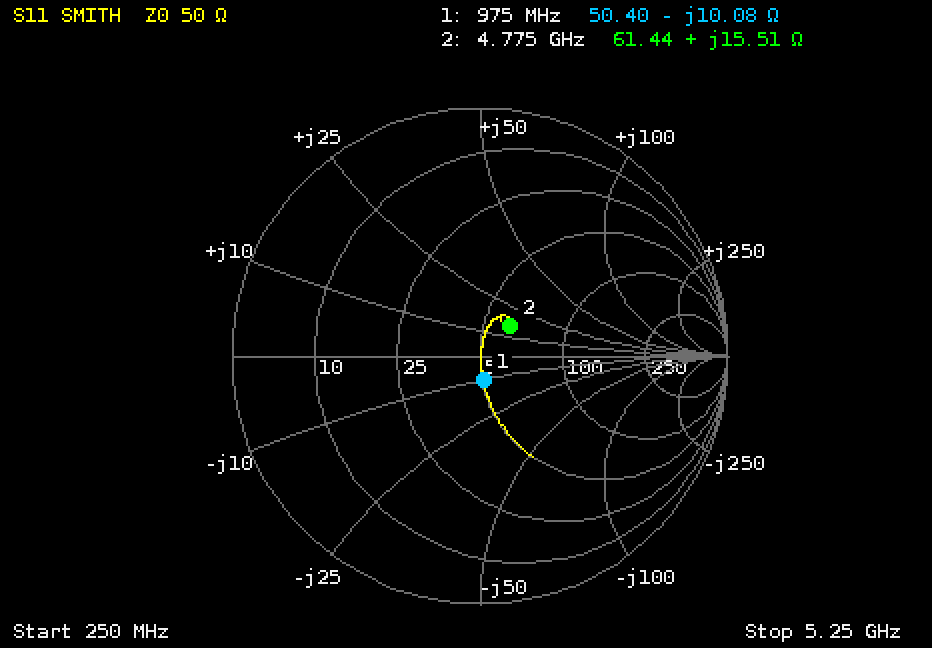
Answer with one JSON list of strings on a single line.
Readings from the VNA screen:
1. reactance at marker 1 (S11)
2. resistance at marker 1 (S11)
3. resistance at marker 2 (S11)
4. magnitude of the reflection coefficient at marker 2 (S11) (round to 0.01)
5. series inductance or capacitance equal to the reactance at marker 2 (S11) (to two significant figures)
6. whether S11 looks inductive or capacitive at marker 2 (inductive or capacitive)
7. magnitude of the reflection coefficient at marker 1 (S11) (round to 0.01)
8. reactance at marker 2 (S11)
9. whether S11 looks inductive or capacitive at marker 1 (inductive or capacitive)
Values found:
["-10.08 Ω", "50.40 Ω", "61.44 Ω", "0.17", "520 pH", "inductive", "0.10", "+15.51 Ω", "capacitive"]
